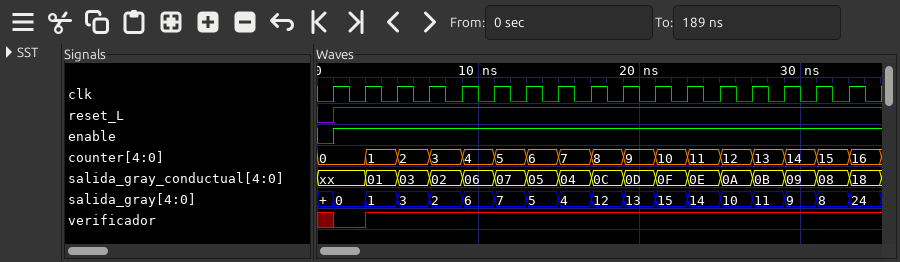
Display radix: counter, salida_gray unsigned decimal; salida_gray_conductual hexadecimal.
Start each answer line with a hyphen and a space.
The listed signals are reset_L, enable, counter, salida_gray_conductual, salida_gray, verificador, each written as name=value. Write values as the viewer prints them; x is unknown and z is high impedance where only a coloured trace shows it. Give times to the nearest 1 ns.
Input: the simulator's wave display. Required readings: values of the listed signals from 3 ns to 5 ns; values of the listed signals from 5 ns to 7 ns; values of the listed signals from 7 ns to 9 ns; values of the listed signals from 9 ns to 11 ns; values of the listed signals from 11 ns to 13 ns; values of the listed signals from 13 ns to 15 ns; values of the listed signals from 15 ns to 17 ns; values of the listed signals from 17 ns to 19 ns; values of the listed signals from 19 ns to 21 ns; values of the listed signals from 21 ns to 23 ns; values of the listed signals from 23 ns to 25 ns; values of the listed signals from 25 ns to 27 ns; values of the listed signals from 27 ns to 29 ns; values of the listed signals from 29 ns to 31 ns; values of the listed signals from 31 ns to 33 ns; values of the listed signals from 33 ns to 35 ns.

- reset_L=1, enable=1, counter=1, salida_gray_conductual=01, salida_gray=1, verificador=1
- reset_L=1, enable=1, counter=2, salida_gray_conductual=03, salida_gray=3, verificador=1
- reset_L=1, enable=1, counter=3, salida_gray_conductual=02, salida_gray=2, verificador=1
- reset_L=1, enable=1, counter=4, salida_gray_conductual=06, salida_gray=6, verificador=1
- reset_L=1, enable=1, counter=5, salida_gray_conductual=07, salida_gray=7, verificador=1
- reset_L=1, enable=1, counter=6, salida_gray_conductual=05, salida_gray=5, verificador=1
- reset_L=1, enable=1, counter=7, salida_gray_conductual=04, salida_gray=4, verificador=1
- reset_L=1, enable=1, counter=8, salida_gray_conductual=0C, salida_gray=12, verificador=1
- reset_L=1, enable=1, counter=9, salida_gray_conductual=0D, salida_gray=13, verificador=1
- reset_L=1, enable=1, counter=10, salida_gray_conductual=0F, salida_gray=15, verificador=1
- reset_L=1, enable=1, counter=11, salida_gray_conductual=0E, salida_gray=14, verificador=1
- reset_L=1, enable=1, counter=12, salida_gray_conductual=0A, salida_gray=10, verificador=1
- reset_L=1, enable=1, counter=13, salida_gray_conductual=0B, salida_gray=11, verificador=1
- reset_L=1, enable=1, counter=14, salida_gray_conductual=09, salida_gray=9, verificador=1
- reset_L=1, enable=1, counter=15, salida_gray_conductual=08, salida_gray=8, verificador=1
- reset_L=1, enable=1, counter=16, salida_gray_conductual=18, salida_gray=24, verificador=1
